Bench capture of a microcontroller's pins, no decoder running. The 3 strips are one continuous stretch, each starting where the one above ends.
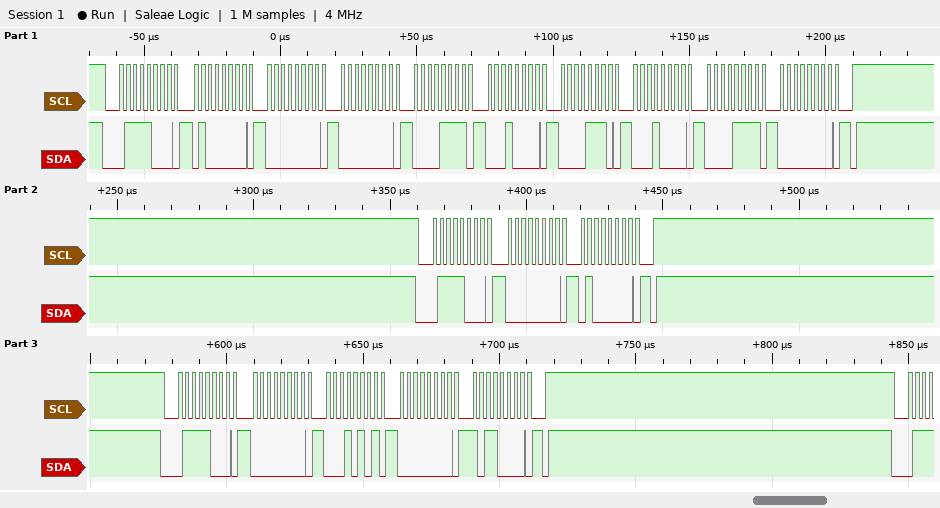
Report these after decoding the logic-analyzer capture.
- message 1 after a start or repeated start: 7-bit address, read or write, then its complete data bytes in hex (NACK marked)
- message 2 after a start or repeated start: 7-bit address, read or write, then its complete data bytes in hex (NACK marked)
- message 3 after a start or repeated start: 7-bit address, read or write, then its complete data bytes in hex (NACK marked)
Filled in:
0x3C write: 40 00 00 0F 10 0E 10 0F 00
0x3C write: 00 40
0x3C write: 00 15 00 B0
